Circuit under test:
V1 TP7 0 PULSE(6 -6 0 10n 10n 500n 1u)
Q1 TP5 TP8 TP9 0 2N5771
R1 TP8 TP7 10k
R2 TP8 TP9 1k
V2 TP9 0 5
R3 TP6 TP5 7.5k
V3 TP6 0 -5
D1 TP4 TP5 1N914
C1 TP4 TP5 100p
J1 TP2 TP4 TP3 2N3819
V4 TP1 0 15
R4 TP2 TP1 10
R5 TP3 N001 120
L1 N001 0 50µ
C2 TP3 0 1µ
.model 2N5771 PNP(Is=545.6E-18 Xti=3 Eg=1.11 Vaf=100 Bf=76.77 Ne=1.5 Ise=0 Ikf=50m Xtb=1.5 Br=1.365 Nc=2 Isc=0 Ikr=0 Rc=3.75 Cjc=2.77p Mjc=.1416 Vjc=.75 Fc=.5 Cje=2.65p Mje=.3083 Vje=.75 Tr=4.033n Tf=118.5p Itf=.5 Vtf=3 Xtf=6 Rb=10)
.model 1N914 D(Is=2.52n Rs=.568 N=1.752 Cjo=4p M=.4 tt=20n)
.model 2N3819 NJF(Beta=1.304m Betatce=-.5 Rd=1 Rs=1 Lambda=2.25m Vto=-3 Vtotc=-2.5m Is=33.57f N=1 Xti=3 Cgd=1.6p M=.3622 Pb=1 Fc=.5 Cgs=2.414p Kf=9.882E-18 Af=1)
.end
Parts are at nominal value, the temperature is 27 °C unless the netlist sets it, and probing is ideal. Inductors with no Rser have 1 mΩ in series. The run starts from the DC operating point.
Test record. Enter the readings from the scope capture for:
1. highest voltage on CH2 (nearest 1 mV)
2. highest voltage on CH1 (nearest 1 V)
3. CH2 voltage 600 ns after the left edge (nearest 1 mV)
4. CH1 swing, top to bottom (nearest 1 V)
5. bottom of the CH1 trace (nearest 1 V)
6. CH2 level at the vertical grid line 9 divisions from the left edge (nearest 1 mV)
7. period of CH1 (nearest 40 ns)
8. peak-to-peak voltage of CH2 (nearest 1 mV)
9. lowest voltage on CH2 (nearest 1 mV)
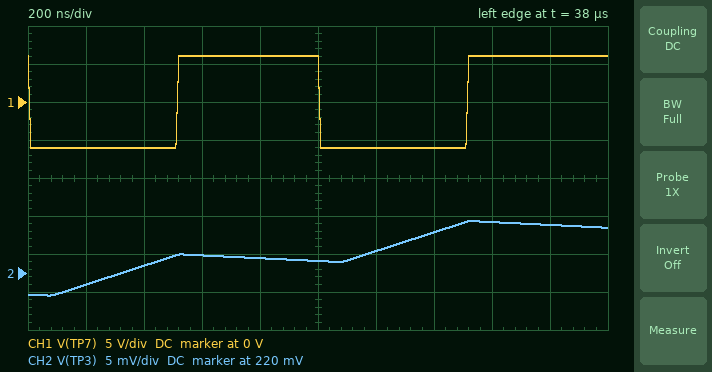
227 mV
6 V
222 mV
12 V
-6 V
226 mV
1.00 µs
10 mV
217 mV
